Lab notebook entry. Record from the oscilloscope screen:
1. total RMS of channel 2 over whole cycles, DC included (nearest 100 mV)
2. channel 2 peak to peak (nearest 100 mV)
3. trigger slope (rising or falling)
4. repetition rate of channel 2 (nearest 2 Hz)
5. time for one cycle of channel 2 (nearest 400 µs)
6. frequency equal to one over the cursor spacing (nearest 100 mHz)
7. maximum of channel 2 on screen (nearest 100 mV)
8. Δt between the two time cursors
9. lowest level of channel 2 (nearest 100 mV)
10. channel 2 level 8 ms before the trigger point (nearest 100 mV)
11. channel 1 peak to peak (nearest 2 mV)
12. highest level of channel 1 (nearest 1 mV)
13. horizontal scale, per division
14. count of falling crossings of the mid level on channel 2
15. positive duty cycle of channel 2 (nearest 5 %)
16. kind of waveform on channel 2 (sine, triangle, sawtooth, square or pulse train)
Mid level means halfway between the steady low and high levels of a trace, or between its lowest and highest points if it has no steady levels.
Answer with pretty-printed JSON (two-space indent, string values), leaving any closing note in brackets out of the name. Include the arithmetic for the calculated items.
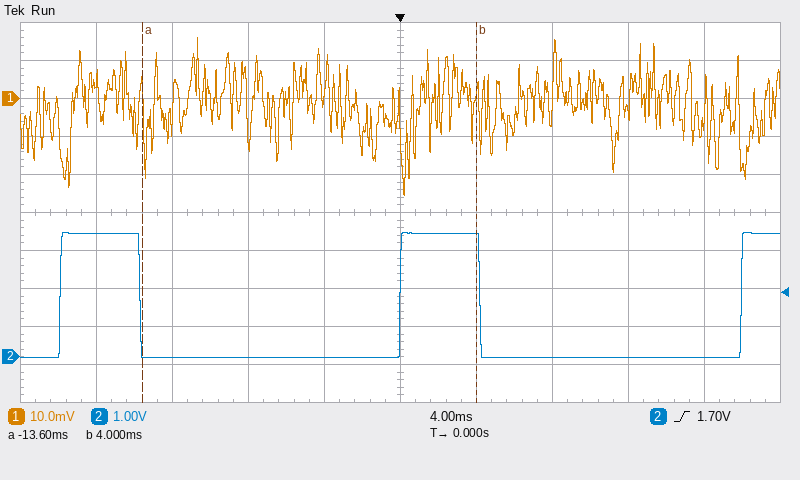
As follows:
{
  "total RMS of channel 2 over whole cycles, DC included": "√(0.25 × (3.3 V)² + 0.75 × (0.0 V)²) ≈ 1.6 V",
  "channel 2 peak to peak": "3.3 V − (0.0 V) = 3.3 V",
  "trigger slope": "rising",
  "repetition rate of channel 2": "1 / 18.0 ms ≈ 56 Hz",
  "time for one cycle of channel 2": "18.0 ms",
  "frequency equal to one over the cursor spacing": "1 / 17.6 ms ≈ 56.8 Hz",
  "maximum of channel 2 on screen": "3.3 V",
  "Δt between the two time cursors": "4 ms − (-13.6 ms) = 17.6 ms",
  "lowest level of channel 2": "0.0 V",
  "channel 2 level 8 ms before the trigger point": "0.0 V",
  "channel 1 peak to peak": "42 mV",
  "highest level of channel 1": "16 mV",
  "horizontal scale, per division": "4 ms",
  "count of falling crossings of the mid level on channel 2": "2",
  "positive duty cycle of channel 2": "25 %",
  "kind of waveform on channel 2": "pulse train"
}
